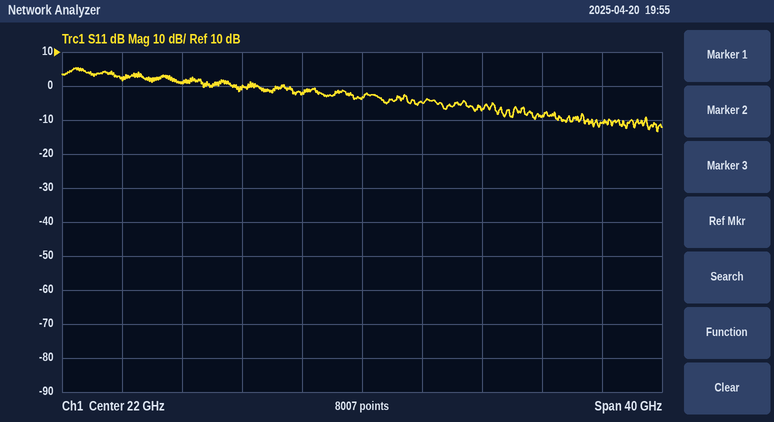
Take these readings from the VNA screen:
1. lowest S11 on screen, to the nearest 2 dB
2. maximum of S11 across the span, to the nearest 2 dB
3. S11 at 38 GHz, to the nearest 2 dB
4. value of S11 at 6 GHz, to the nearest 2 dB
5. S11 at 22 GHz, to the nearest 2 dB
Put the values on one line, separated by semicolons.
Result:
-14 dB; 6 dB; -10 dB; 2 dB; -4 dB
